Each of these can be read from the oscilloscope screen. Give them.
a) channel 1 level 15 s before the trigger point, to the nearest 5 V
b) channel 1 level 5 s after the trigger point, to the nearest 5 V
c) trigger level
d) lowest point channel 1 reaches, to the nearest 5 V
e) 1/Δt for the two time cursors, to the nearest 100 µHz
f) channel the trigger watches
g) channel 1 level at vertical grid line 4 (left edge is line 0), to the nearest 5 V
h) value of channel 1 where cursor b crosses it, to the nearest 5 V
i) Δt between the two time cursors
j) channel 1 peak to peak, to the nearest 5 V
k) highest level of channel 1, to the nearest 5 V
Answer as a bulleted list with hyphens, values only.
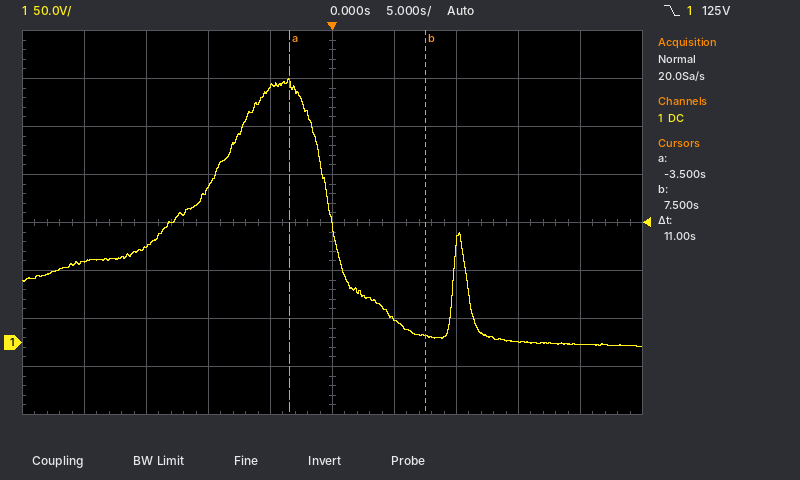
- 100 V
- 25 V
- 125 V
- -5 V
- 90.9 mHz
- channel 1
- 265 V
- 5 V
- 11 s
- 280 V
- 275 V
